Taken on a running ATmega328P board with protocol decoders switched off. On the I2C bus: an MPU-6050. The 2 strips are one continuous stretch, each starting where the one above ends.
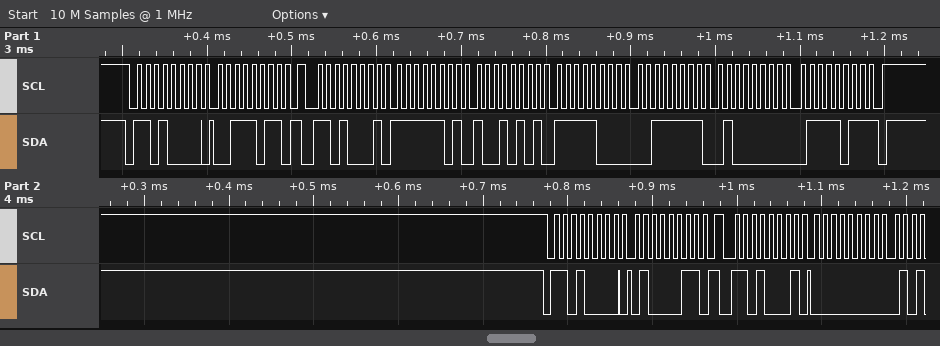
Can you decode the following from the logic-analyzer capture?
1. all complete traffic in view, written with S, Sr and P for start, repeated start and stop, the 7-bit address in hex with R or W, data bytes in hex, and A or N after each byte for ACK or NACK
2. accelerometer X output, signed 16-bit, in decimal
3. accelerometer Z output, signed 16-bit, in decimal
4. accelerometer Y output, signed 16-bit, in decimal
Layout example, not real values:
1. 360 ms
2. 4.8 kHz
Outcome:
1. S 68W A 3B A Sr 68R A FD A 95 A F8 A 3F A 40 A 7B N P S 68W A 43 A Sr 68R A 00 A
2. -619
3. 16507
4. -1985
